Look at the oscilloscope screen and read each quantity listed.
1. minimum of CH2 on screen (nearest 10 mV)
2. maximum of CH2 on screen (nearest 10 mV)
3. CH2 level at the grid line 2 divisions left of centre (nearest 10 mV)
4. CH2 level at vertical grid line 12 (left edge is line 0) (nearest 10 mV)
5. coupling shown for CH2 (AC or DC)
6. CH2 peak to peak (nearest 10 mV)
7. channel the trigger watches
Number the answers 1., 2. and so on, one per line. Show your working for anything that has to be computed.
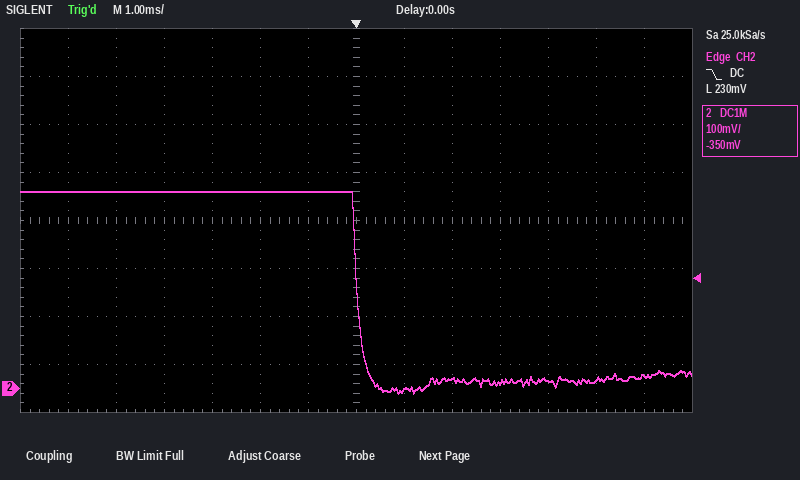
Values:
1. -10 mV
2. 410 mV
3. 410 mV
4. 20 mV
5. DC
6. 410 mV − (-10 mV) = 420 mV
7. CH2
